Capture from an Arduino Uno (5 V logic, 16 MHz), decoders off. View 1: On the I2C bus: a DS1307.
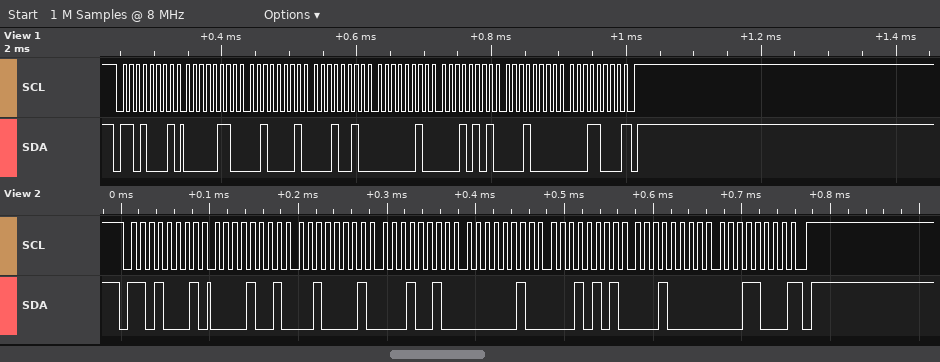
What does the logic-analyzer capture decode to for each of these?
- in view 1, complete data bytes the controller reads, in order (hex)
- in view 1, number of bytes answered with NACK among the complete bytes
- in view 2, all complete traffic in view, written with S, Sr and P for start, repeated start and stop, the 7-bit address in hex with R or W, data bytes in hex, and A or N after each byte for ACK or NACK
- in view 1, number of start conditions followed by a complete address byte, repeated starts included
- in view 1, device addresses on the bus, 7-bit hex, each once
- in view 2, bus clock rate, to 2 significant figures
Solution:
06 21 12 02 15 10 18
1
S 68R A 09 A 21 A 12 A 02 A 15 A 10 A 18 N P
1
0x68
100 kHz
